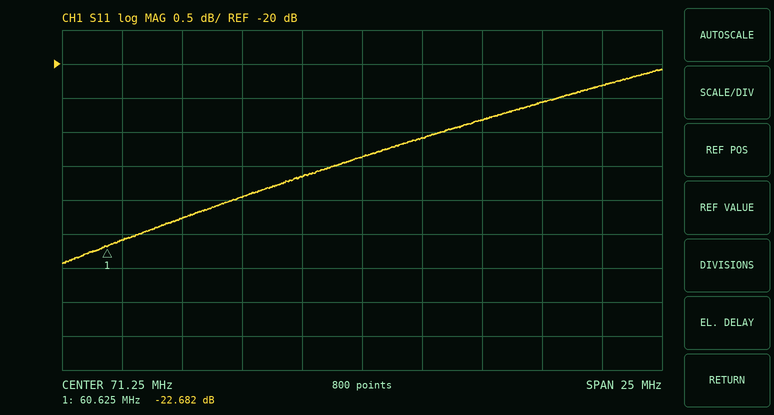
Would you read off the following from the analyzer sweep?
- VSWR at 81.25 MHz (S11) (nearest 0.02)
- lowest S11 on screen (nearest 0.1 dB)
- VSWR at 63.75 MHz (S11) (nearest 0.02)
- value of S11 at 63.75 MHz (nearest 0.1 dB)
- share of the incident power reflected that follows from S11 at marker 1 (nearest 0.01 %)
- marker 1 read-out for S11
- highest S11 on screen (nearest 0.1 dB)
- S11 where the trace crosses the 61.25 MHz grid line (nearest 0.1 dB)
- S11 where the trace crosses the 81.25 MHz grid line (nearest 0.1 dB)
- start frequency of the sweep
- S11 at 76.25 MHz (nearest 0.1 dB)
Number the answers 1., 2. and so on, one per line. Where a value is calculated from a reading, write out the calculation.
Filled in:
1. |Γ| = 10^(-20.3/20) = 0.0966; VSWR = (1 + 0.0966)/(1 − 0.0966) ≈ 1.21, so 1.22 to the nearest 0.02
2. -22.9 dB
3. |Γ| = 10^(-22.3/20) = 0.0767; VSWR = (1 + 0.0767)/(1 − 0.0767) ≈ 1.17, so 1.16 to the nearest 0.02
4. -22.3 dB
5. 10^(-22.682/10) ≈ 0.54 %
6. -22.682 dB
7. -20.1 dB
8. -22.6 dB
9. -20.3 dB
10. 58.75 MHz
11. -20.8 dB
